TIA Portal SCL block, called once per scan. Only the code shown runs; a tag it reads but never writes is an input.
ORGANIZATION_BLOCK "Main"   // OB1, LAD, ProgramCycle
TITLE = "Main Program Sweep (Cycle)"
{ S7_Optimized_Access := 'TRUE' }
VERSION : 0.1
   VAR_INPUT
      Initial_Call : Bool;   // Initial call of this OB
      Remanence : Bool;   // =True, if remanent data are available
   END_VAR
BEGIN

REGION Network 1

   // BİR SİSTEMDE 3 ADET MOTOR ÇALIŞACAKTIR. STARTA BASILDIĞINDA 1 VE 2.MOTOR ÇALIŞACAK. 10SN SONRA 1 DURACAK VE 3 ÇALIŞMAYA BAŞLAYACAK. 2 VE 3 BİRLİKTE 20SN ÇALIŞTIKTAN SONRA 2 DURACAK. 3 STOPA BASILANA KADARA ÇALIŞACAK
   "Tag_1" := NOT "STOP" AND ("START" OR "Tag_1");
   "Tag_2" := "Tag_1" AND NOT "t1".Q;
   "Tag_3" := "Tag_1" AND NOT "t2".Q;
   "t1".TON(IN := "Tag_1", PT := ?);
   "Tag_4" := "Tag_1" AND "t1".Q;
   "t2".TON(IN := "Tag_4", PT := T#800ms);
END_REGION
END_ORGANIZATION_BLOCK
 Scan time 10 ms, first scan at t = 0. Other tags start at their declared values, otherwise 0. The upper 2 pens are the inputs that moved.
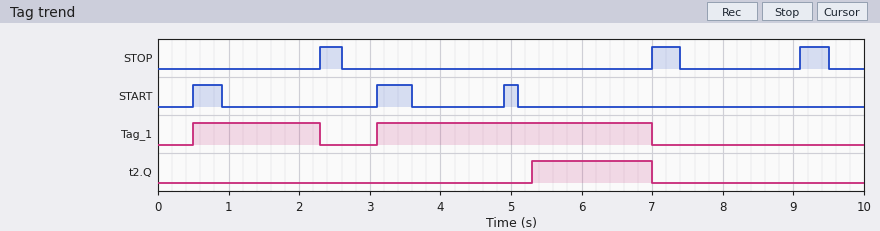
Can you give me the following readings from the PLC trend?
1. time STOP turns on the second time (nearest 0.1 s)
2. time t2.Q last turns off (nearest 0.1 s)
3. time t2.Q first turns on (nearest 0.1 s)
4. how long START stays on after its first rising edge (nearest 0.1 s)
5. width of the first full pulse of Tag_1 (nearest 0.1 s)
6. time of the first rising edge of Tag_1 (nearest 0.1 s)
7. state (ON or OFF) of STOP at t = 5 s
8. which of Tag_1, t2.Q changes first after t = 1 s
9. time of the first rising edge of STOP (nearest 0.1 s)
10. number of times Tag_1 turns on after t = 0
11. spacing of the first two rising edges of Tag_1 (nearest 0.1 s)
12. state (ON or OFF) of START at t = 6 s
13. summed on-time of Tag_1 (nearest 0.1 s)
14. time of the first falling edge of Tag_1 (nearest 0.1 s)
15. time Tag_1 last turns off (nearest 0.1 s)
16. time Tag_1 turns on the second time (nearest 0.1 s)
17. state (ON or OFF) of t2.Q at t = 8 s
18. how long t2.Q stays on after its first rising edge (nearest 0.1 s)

7.0 s
7.0 s
5.3 s
0.4 s
1.8 s
0.5 s
OFF
Tag_1
2.3 s
2
2.6 s
OFF
5.7 s
2.3 s
7.0 s
3.1 s
OFF
1.7 s
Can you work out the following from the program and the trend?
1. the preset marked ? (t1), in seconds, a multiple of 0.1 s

1.4 s
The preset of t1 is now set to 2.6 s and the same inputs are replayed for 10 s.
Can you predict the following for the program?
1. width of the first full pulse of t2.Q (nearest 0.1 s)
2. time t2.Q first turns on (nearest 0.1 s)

0.5 s
6.5 s
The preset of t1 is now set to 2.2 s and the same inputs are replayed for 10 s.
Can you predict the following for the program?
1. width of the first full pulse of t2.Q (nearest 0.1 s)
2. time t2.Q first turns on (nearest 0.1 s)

0.9 s
6.1 s
